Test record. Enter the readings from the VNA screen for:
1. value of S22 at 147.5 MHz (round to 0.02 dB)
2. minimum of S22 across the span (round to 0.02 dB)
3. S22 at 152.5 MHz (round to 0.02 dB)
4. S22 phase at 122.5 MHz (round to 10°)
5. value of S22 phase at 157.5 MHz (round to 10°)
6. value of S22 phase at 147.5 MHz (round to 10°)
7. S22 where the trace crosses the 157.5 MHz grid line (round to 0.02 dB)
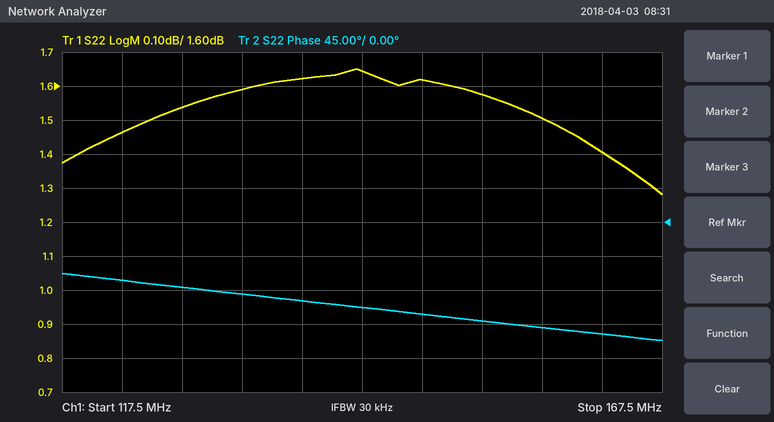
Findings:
1.62 dB
1.28 dB
1.58 dB
-80°
-140°
-120°
1.50 dB
